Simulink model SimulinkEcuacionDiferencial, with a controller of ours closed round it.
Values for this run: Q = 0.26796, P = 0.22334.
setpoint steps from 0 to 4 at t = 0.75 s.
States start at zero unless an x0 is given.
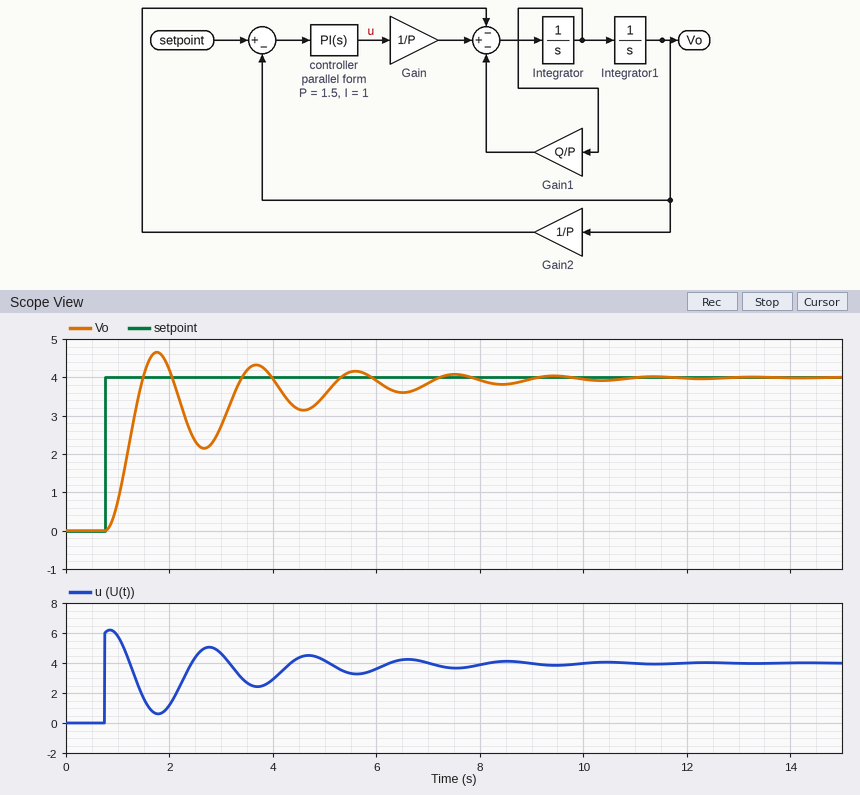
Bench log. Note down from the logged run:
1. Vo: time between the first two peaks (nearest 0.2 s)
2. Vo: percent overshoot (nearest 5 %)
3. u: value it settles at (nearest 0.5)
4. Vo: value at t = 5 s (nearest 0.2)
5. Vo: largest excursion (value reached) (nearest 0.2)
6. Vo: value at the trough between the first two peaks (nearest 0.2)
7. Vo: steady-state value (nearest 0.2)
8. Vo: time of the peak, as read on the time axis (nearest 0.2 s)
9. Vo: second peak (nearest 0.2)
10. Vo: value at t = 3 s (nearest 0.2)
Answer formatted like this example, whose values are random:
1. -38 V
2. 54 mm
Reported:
1. 2.0 s
2. 15 %
3. 4.0
4. 3.6
5. 4.6
6. 2.2
7. 4.0
8. 1.8 s
9. 4.4
10. 2.8
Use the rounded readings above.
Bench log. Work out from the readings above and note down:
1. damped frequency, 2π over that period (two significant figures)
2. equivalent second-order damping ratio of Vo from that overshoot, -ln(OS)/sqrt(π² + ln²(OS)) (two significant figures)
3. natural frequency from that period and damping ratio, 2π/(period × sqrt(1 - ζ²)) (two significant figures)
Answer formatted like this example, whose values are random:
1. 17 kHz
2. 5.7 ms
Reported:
1. 3.1 rad/s
2. 0.52
3. 3.7 rad/s
